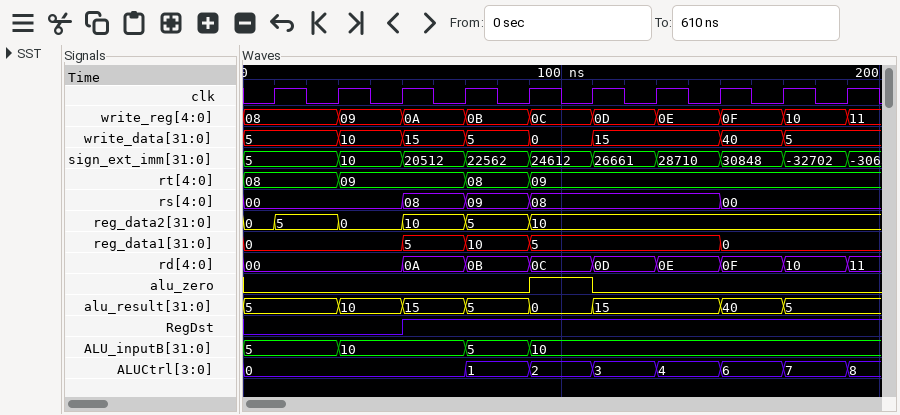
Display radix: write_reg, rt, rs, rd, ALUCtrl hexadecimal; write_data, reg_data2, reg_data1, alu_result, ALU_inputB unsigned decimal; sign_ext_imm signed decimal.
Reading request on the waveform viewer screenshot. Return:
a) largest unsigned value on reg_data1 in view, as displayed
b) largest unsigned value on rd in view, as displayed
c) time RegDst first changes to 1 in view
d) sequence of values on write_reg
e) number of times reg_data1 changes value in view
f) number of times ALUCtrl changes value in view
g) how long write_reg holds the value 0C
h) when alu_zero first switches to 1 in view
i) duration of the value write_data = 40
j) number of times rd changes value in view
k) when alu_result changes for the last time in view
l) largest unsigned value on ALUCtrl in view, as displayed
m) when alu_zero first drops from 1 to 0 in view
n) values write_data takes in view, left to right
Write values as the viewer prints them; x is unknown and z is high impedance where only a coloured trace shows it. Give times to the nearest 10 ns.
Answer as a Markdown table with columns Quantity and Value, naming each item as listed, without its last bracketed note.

| Quantity | Value |
|---|---|
| largest unsigned value on reg_data1 in view, as displayed | 10 |
| largest unsigned value on rd in view, as displayed | 11 |
| time RegDst first changes to 1 in view | 50 ns |
| sequence of values on write_reg | 08, 09, 0A, 0B, 0C, 0D, 0E, 0F, 10, 11 |
| number of times reg_data1 changes value in view | 4 |
| number of times ALUCtrl changes value in view | 7 |
| how long write_reg holds the value 0C | 20 ns |
| when alu_zero first switches to 1 in view | 90 ns |
| duration of the value write_data = 40 | 20 ns |
| number of times rd changes value in view | 8 |
| when alu_result changes for the last time in view | 170 ns |
| largest unsigned value on ALUCtrl in view, as displayed | 8 |
| when alu_zero first drops from 1 to 0 in view | 110 ns |
| values write_data takes in view, left to right | 5, 10, 15, 5, 0, 15, 40, 5 |
